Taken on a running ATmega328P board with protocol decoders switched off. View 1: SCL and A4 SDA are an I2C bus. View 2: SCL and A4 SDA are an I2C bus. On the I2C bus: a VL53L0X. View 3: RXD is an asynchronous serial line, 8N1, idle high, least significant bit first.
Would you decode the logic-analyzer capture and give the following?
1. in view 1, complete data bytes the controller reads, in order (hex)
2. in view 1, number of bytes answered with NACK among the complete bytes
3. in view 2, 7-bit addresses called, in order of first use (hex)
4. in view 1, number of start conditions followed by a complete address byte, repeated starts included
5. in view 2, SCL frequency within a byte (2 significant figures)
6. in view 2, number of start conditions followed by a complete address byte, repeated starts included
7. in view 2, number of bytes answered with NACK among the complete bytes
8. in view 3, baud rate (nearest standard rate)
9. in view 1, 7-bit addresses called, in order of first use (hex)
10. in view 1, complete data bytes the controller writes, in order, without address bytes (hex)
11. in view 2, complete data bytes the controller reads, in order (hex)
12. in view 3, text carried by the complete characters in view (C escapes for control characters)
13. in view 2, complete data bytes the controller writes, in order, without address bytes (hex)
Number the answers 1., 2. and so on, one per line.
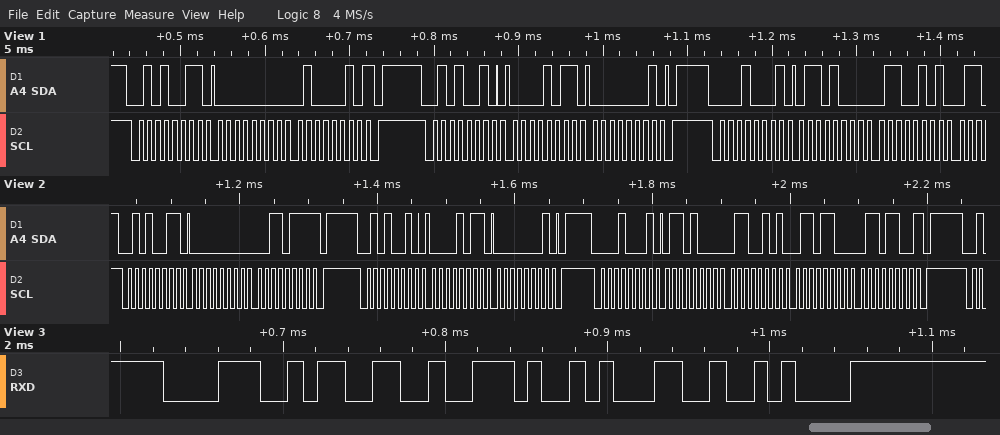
1. 00 42 68 65
2. 1
3. 0x29 0x08
4. 3
5. 100 kHz
6. 3
7. 2
8. 115200 baud
9. 0x29 0x08
10. 0B 01
11. 00 37 68 65 6C 6C
12. "83.1\n"
13. 0B 01
